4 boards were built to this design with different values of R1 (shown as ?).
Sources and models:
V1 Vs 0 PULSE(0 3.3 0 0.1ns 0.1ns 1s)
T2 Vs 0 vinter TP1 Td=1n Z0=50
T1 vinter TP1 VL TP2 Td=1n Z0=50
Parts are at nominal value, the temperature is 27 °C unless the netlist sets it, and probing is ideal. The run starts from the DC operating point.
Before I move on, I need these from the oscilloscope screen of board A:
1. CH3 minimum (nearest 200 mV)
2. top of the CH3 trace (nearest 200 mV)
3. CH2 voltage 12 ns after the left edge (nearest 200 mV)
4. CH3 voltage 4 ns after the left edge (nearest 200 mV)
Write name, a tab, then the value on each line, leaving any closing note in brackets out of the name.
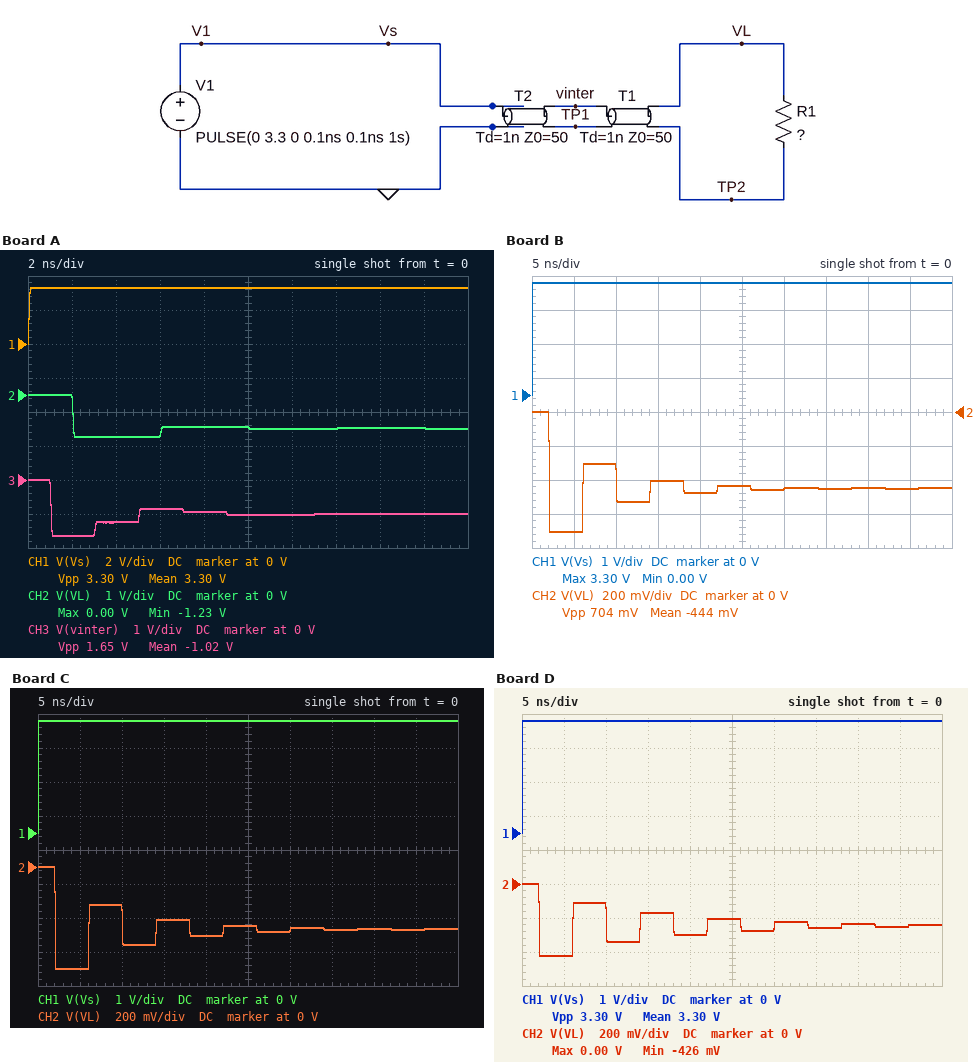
CH3 minimum	-1.6 V
top of the CH3 trace	0 V
CH2 voltage 12 ns after the left edge	-1.0 V
CH3 voltage 4 ns after the left edge	-1.2 V
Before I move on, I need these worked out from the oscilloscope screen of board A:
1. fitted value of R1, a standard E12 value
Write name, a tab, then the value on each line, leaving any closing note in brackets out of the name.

fitted value of R1, a standard E12 value	82 Ω
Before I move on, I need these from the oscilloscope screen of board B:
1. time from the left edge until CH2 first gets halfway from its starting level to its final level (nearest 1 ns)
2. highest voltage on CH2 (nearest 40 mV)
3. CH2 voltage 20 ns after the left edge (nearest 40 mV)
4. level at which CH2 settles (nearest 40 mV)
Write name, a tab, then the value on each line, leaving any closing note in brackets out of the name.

time from the left edge until CH2 first gets halfway from its starting level to its final level	2 ns
highest voltage on CH2	0 V
CH2 voltage 20 ns after the left edge	-480 mV
level at which CH2 settles	-440 mV
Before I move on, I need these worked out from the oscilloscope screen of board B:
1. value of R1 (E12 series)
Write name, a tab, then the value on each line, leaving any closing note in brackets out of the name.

value of R1	180 Ω
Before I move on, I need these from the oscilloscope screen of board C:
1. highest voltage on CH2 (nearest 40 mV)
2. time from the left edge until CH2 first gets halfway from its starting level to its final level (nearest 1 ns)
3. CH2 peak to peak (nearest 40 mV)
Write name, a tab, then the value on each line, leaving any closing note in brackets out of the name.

highest voltage on CH2	0 V
time from the left edge until CH2 first gets halfway from its starting level to its final level	2 ns
CH2 peak to peak	600 mV
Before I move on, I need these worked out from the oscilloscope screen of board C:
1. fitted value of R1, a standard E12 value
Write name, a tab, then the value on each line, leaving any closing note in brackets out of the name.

fitted value of R1, a standard E12 value	220 Ω
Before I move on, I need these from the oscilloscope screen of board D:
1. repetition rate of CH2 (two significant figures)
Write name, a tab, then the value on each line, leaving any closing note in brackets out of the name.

repetition rate of CH2	120 MHz
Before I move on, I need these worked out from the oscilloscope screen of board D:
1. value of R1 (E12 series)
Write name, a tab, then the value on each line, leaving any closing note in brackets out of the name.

value of R1	330 Ω
